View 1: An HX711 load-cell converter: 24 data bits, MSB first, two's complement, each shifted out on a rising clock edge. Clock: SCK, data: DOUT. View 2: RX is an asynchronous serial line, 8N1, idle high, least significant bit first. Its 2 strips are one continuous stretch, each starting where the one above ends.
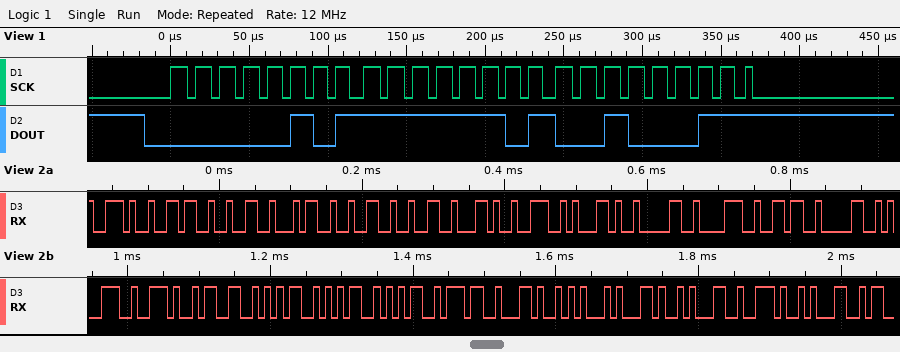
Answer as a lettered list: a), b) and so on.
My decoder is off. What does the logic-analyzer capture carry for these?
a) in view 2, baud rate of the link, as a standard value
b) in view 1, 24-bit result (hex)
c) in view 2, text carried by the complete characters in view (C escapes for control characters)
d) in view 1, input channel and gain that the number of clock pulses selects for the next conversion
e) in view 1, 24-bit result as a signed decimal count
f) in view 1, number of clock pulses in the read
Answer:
a) 115200 baud
b) 0x05FD23
c) ".62422,N,08609.35557,E,1.1"
d) channel A, gain 128
e) 392483
f) 25
